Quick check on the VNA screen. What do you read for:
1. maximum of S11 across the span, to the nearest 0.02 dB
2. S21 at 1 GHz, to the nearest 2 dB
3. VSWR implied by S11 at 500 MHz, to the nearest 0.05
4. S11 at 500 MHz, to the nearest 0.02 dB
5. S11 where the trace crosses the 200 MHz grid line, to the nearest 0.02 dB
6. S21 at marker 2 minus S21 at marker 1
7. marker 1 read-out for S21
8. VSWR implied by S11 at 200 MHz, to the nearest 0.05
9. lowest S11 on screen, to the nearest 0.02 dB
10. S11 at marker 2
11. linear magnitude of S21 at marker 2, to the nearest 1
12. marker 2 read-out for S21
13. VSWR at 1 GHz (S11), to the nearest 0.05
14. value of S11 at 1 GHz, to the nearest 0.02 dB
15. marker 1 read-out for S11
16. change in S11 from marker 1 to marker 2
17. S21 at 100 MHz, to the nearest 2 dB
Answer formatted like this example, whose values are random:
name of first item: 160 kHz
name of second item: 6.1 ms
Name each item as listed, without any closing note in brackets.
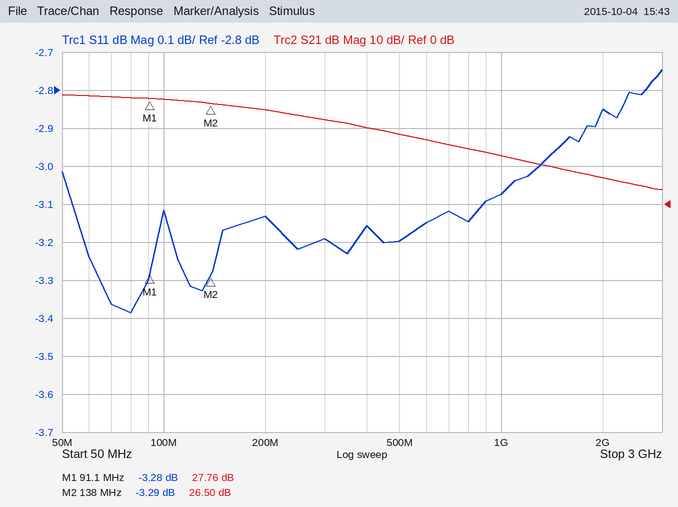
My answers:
maximum of S11 across the span, to the nearest 0.02 dB: -2.74 dB
S21 at 1 GHz, to the nearest 2 dB: 12 dB
VSWR implied by S11 at 500 MHz, to the nearest 0.05: 5.50
S11 at 500 MHz, to the nearest 0.02 dB: -3.20 dB
S11 where the trace crosses the 200 MHz grid line, to the nearest 0.02 dB: -3.14 dB
S21 at marker 2 minus S21 at marker 1: -1.26 dB
marker 1 read-out for S21: 27.76 dB
VSWR implied by S11 at 200 MHz, to the nearest 0.05: 5.60
lowest S11 on screen, to the nearest 0.02 dB: -3.38 dB
S11 at marker 2: -3.29 dB
linear magnitude of S21 at marker 2, to the nearest 1: 21
marker 2 read-out for S21: 26.50 dB
VSWR at 1 GHz (S11), to the nearest 0.05: 5.70
value of S11 at 1 GHz, to the nearest 0.02 dB: -3.08 dB
marker 1 read-out for S11: -3.28 dB
change in S11 from marker 1 to marker 2: -0.01 dB
S21 at 100 MHz, to the nearest 2 dB: 28 dB
